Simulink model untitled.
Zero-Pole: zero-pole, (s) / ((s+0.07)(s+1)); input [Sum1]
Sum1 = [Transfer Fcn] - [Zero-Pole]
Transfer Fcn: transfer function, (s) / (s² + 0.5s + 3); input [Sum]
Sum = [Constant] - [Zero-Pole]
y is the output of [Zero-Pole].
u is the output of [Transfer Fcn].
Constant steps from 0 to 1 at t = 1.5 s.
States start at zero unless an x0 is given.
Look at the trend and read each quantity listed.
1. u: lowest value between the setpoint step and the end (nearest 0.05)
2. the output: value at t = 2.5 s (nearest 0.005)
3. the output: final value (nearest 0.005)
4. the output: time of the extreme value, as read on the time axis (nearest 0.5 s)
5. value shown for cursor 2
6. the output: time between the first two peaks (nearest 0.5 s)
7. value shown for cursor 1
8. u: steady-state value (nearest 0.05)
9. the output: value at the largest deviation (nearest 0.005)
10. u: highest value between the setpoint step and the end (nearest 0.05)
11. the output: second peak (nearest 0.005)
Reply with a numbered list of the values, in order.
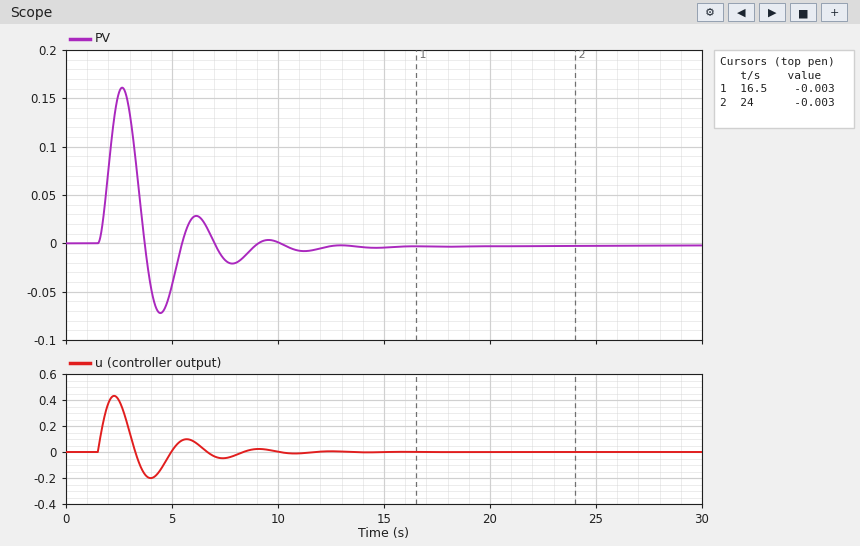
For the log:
1. -0.20
2. 0.155
3. 0.000
4. 2.5 s
5. -0.003
6. 3.5 s
7. -0.003
8. 0.00
9. 0.160
10. 0.45
11. 0.030
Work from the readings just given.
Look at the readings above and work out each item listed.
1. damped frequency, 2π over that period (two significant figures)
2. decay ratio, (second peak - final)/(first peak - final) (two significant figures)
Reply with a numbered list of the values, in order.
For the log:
1. 1.8 rad/s
2. 0.19
